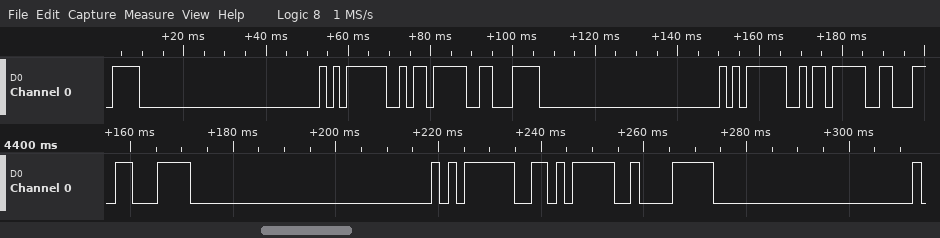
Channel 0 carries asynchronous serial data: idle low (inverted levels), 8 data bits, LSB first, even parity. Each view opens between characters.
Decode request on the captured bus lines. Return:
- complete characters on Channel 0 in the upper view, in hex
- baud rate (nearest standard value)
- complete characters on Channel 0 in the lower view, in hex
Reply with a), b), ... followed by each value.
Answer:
a) F8, 05, 09, 0E, 05, 09
b) 600 baud
c) 0E, 05, 0A, 0F
